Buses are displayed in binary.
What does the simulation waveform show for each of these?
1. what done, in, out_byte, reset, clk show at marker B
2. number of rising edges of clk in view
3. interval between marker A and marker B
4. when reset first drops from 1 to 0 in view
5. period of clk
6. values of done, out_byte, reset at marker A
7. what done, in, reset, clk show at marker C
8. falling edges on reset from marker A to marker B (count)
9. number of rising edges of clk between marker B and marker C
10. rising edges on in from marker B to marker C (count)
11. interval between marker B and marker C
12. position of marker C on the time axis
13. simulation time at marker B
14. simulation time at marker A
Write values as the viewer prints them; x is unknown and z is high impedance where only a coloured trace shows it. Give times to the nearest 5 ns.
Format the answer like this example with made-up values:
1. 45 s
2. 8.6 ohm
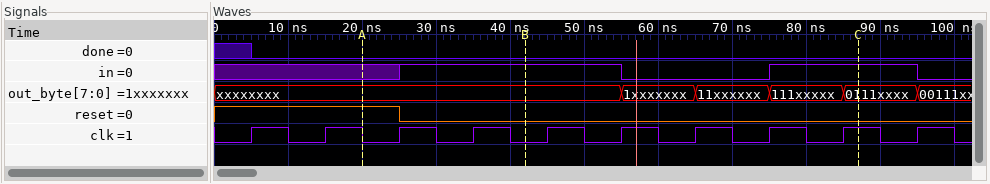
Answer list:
1. done=0, in=1, out_byte=xxxxxxxx, reset=0, clk=0
2. 10
3. 20 ns
4. 25 ns
5. 10 ns
6. done=0, out_byte=xxxxxxxx, reset=1
7. done=0, in=1, reset=0, clk=1
8. 1
9. 5
10. 1
11. 45 ns
12. 85 ns
13. 40 ns
14. 20 ns
